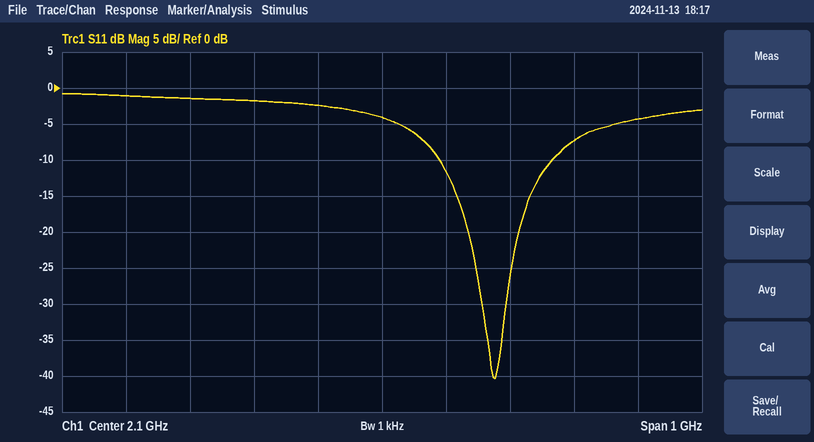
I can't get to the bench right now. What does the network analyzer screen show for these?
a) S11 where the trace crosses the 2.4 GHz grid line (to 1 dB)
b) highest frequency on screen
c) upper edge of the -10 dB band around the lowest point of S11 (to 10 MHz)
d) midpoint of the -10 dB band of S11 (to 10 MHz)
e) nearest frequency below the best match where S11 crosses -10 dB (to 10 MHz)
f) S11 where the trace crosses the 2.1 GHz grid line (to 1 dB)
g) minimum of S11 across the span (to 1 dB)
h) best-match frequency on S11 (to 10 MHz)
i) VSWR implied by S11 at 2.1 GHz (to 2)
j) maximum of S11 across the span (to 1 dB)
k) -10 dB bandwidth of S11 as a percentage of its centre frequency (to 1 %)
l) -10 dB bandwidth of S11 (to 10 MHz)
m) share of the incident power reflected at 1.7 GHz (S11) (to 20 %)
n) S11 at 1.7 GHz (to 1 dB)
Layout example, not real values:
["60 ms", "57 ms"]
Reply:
["-7 dB", "2.6 GHz", "2.37 GHz", "2.28 GHz", "2.19 GHz", "-4 dB", "-40 dB", "2.28 GHz", "4", "-1 dB", "8 %", "180 MHz", "80 %", "-1 dB"]
